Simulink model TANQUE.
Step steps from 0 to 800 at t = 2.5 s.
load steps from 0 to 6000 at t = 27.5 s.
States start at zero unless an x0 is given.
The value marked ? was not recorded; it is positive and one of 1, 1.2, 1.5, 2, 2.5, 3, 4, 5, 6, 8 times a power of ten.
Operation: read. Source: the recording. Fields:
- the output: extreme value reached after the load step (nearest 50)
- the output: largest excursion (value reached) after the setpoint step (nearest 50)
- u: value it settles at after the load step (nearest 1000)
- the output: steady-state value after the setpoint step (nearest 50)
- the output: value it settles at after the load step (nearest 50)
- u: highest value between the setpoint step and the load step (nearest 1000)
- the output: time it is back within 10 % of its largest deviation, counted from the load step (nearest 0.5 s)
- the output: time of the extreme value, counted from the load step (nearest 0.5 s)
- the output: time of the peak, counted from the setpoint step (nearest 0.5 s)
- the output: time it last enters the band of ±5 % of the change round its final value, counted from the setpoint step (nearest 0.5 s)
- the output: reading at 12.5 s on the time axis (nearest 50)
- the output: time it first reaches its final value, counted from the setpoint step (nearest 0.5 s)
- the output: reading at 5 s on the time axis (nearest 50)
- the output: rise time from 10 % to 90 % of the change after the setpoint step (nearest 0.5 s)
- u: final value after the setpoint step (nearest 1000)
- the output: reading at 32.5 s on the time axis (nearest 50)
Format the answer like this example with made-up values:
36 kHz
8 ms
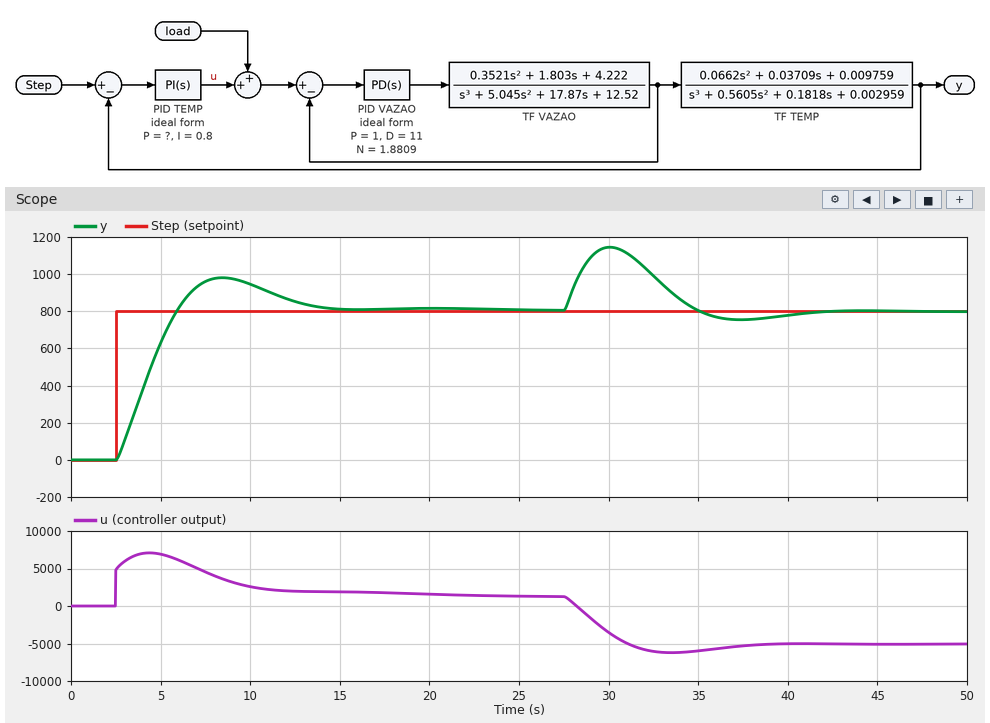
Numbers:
1150
1000
-5000
800
800
7000
11.5 s
2.5 s
6.0 s
10.5 s
850
3.5 s
650
2.5 s
1000
1000
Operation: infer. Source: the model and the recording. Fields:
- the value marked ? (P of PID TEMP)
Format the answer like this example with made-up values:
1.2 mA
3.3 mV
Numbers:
6
